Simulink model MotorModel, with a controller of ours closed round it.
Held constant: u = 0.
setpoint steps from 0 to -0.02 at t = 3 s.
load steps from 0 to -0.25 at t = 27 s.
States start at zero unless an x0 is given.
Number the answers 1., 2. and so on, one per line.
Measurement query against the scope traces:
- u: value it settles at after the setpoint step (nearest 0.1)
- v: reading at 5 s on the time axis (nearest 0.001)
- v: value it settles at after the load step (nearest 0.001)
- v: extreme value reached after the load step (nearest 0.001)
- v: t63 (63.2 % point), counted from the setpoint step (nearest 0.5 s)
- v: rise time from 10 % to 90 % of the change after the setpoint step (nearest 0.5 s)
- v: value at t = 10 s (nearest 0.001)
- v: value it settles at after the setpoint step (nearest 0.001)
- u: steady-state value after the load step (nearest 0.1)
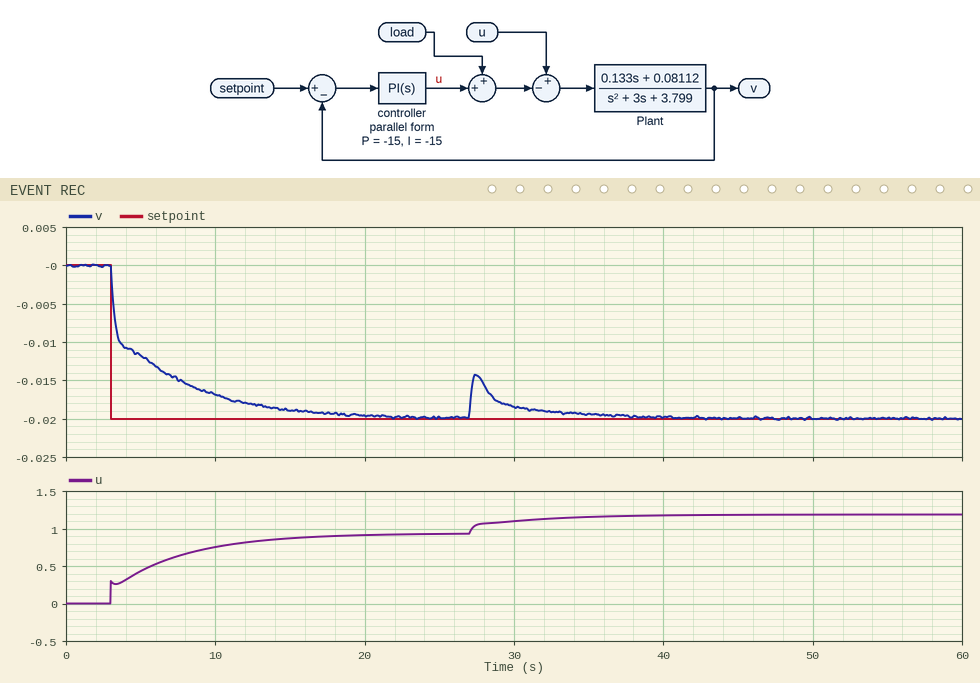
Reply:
1. 0.9
2. -0.012
3. -0.020
4. -0.014
5. 2.5 s
6. 9.0 s
7. -0.017
8. -0.020
9. 1.2
